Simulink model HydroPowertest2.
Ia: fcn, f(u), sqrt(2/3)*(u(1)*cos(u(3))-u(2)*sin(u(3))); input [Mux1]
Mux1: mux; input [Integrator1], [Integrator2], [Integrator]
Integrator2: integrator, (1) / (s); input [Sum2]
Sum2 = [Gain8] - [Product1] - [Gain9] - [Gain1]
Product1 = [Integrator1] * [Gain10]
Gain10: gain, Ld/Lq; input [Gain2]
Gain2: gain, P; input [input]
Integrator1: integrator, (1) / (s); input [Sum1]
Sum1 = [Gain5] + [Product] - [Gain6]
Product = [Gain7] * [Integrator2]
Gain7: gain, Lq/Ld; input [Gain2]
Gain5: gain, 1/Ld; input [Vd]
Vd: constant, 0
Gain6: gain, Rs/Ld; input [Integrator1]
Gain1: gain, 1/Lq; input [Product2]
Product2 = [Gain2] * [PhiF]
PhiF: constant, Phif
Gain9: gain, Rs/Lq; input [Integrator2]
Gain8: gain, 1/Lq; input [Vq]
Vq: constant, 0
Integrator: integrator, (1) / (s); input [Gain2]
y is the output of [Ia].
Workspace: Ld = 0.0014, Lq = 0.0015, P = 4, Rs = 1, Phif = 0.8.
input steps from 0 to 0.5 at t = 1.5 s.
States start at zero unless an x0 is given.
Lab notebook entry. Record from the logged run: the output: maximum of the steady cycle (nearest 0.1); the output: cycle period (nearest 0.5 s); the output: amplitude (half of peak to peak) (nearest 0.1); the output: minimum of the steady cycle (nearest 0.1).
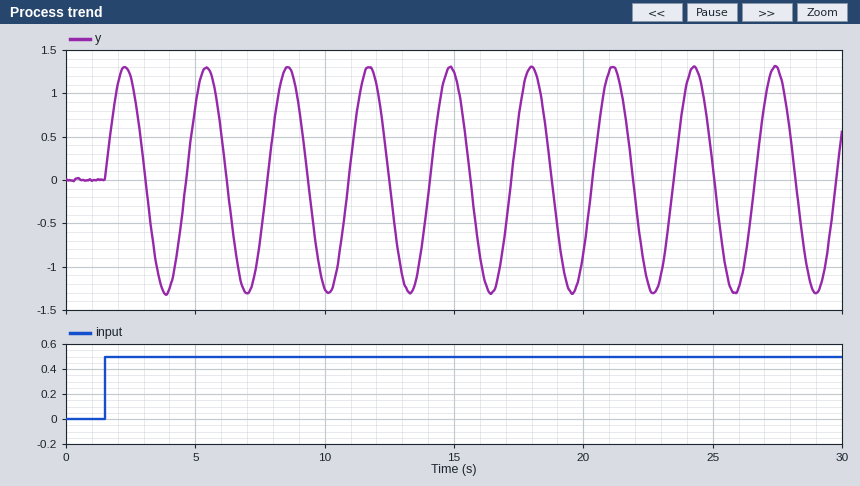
1.3
3.0 s
1.3
-1.3
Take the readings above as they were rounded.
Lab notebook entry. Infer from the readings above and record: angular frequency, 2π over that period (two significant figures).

2.1 rad/s
